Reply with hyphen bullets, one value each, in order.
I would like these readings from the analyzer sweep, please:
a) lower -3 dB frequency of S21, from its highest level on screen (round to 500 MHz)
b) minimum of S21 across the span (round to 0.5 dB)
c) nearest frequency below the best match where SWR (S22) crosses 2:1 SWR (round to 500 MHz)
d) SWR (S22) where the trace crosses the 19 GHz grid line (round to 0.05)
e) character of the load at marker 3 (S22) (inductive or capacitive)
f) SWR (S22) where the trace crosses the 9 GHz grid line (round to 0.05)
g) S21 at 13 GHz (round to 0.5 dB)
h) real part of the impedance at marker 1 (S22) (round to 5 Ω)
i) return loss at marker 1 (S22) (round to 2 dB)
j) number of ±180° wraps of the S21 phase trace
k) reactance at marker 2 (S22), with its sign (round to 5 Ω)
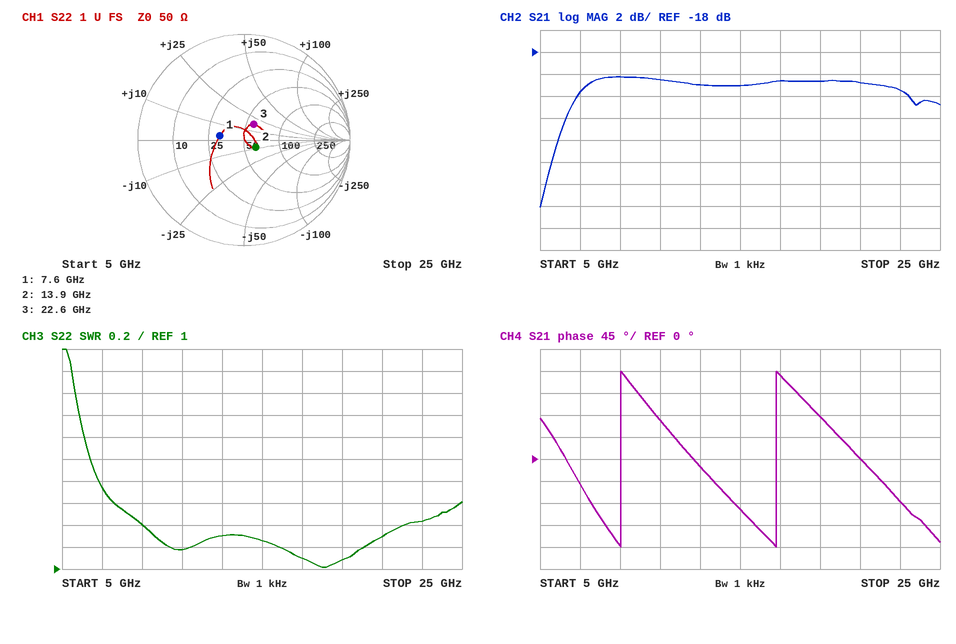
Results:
- 6.5 GHz
- -32.0 dB
- 6.5 GHz
- 1.10
- inductive
- 1.40
- -21.0 dB
- 30 Ω
- 12 dB
- 2
- -10 Ω
